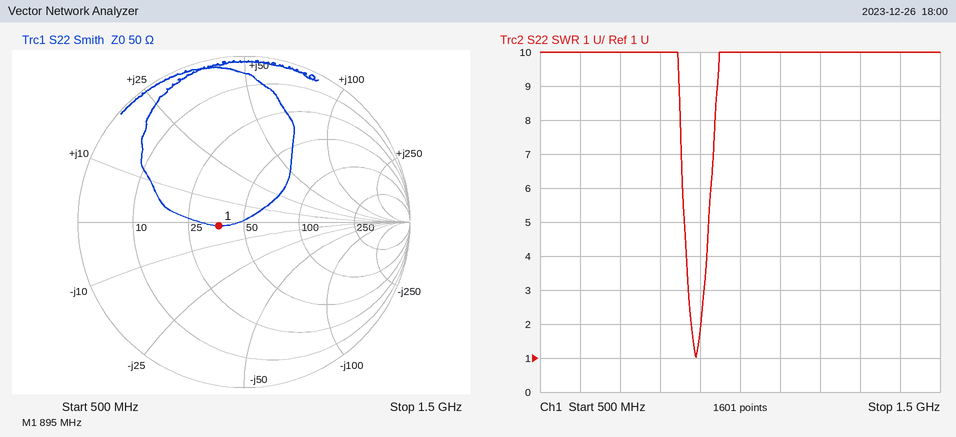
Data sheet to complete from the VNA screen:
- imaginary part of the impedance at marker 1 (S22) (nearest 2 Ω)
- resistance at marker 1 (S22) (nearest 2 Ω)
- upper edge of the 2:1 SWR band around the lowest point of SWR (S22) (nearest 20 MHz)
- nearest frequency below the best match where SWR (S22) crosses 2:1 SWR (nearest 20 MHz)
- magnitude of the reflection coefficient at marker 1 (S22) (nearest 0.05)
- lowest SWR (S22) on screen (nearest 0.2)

-2 Ω
36 Ω
900 MHz
880 MHz
0.15
1.0
